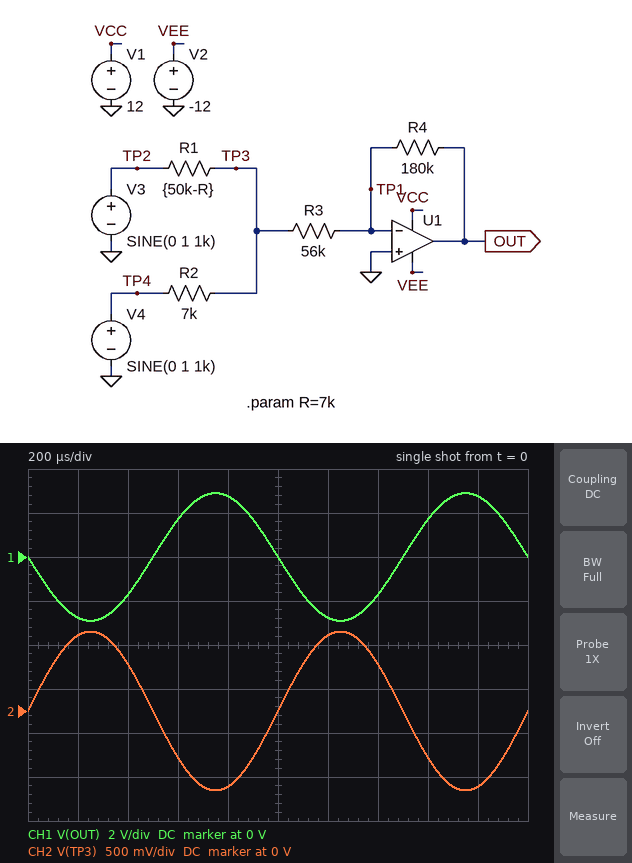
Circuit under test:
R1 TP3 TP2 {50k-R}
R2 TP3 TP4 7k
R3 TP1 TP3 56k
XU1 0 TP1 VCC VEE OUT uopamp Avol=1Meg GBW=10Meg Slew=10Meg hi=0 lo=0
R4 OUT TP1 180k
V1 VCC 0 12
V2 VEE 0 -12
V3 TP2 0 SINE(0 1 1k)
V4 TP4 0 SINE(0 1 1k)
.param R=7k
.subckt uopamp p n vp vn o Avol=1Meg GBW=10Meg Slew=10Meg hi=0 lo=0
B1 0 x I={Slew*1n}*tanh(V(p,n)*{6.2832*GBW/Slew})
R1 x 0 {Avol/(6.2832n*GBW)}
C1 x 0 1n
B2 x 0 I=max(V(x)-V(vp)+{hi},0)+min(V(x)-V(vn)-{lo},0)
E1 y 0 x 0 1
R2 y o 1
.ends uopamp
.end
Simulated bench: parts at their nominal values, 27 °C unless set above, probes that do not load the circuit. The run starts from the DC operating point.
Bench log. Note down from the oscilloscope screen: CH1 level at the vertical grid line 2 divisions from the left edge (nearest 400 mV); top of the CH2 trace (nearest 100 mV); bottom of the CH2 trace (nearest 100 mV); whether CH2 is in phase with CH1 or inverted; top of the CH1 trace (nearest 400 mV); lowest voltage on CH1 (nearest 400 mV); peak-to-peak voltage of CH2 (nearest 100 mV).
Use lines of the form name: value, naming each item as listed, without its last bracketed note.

CH1 level at the vertical grid line 2 divisions from the left edge: -1.6 V
top of the CH2 trace: 900 mV
bottom of the CH2 trace: -900 mV
whether CH2 is in phase with CH1 or inverted: inverted
top of the CH1 trace: 2.8 V
lowest voltage on CH1: -2.8 V
peak-to-peak voltage of CH2: 1.8 V
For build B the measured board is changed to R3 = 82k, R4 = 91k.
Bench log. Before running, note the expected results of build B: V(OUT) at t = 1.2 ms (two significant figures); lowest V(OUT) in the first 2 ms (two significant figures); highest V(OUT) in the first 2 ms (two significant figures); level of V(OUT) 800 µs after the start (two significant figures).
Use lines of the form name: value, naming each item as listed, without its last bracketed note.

V(OUT) at t = 1.2 ms: -980 mV
lowest V(OUT) in the first 2 ms: -1.0 V
highest V(OUT) in the first 2 ms: 1.0 V
level of V(OUT) 800 µs after the start: 980 mV
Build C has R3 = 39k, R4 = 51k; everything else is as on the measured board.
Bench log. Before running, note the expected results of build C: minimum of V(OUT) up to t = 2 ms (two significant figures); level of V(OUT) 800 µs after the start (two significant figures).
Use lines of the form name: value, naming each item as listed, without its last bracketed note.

minimum of V(OUT) up to t = 2 ms: -1.1 V
level of V(OUT) 800 µs after the start: 1.1 V
